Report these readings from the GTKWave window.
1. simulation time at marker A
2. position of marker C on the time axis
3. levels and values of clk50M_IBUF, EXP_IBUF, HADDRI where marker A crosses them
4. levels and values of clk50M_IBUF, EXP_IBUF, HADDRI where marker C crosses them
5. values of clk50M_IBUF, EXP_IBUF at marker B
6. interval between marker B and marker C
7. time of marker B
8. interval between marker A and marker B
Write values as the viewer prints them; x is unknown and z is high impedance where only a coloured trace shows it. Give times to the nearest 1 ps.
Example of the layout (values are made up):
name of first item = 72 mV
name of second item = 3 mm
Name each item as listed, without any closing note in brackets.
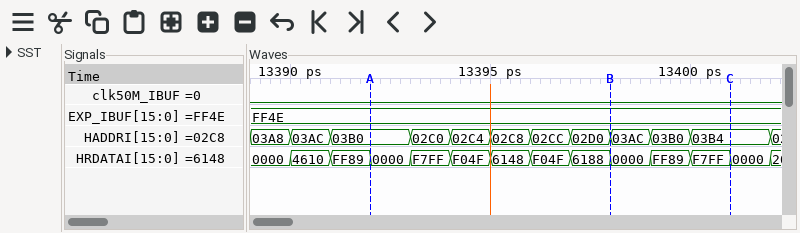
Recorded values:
simulation time at marker A = 13392 ps
position of marker C on the time axis = 13401 ps
levels and values of clk50M_IBUF, EXP_IBUF, HADDRI where marker A crosses them = clk50M_IBUF=0, EXP_IBUF=FF4E, HADDRI=03B0
levels and values of clk50M_IBUF, EXP_IBUF, HADDRI where marker C crosses them = clk50M_IBUF=0, EXP_IBUF=FF4E, HADDRI=03B4
values of clk50M_IBUF, EXP_IBUF at marker B = clk50M_IBUF=0, EXP_IBUF=FF4E
interval between marker B and marker C = 3 ps
time of marker B = 13398 ps
interval between marker A and marker B = 6 ps
